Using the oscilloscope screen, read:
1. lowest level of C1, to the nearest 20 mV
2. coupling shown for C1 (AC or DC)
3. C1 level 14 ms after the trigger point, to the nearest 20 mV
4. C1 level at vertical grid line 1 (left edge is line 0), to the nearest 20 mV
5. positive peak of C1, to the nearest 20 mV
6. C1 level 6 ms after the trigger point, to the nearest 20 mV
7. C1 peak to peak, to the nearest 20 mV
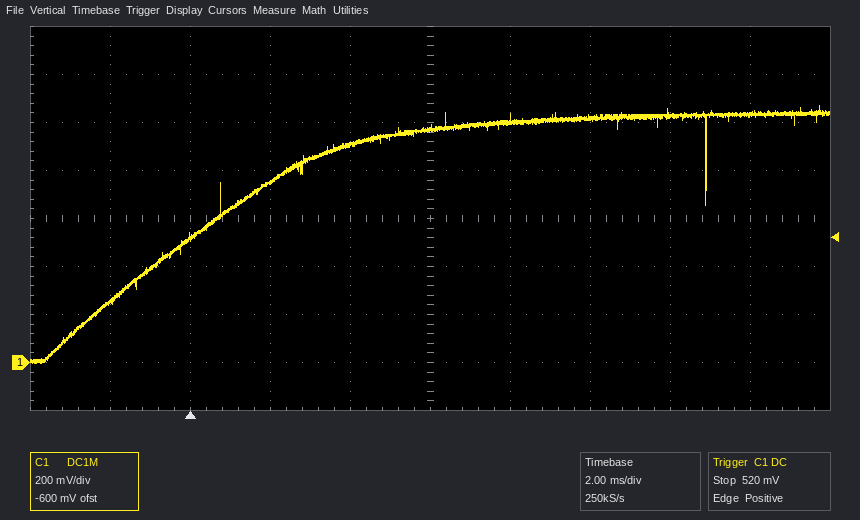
0 mV
DC
1.04 V
260 mV
1.08 V
980 mV
1.08 V
